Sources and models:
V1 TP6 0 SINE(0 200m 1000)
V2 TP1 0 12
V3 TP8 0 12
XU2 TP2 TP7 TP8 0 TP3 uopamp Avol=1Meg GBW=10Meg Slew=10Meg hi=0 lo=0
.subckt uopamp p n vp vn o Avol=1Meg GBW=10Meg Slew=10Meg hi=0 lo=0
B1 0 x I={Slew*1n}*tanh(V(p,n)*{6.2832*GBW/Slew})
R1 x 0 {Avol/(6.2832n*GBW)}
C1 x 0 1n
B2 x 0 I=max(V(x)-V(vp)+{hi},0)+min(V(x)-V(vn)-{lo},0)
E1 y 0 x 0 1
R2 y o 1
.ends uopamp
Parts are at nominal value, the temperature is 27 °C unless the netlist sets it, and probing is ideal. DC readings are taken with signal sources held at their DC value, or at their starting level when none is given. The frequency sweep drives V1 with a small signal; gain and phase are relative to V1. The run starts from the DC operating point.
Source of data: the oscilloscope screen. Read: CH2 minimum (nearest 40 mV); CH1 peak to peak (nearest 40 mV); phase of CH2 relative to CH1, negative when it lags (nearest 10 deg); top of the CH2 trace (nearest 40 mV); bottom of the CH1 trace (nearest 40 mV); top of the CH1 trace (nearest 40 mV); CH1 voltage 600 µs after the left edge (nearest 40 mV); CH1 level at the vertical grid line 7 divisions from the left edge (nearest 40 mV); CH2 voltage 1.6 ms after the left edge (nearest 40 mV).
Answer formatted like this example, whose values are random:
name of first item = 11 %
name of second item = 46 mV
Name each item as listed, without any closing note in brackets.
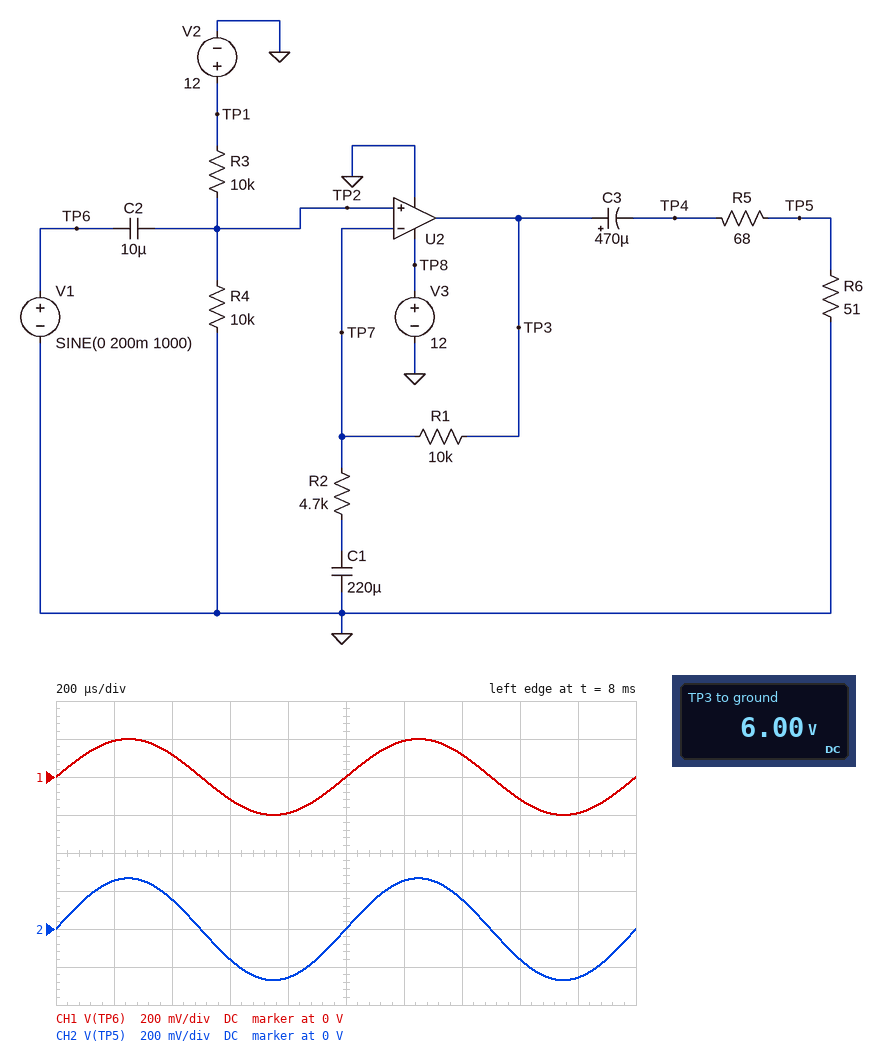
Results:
CH2 minimum = -280 mV
CH1 peak to peak = 400 mV
phase of CH2 relative to CH1, negative when it lags = 0 deg
top of the CH2 trace = 280 mV
bottom of the CH1 trace = -200 mV
top of the CH1 trace = 200 mV
CH1 voltage 600 µs after the left edge = -120 mV
CH1 level at the vertical grid line 7 divisions from the left edge = 120 mV
CH2 voltage 1.6 ms after the left edge = -160 mV
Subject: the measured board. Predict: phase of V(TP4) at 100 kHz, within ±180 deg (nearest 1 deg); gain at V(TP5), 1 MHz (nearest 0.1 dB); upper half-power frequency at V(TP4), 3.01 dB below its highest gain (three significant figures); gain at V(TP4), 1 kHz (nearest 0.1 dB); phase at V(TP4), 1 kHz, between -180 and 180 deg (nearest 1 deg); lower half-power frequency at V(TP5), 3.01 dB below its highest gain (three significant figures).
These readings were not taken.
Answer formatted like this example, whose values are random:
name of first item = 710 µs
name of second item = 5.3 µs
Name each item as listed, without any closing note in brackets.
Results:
phase of V(TP4) at 100 kHz, within ±180 deg = -2 deg
gain at V(TP5), 1 MHz = 2.1 dB
upper half-power frequency at V(TP4), 3.01 dB below its highest gain = 3.17 MHz
gain at V(TP4), 1 kHz = 9.9 dB
phase at V(TP4), 1 kHz, between -180 and 180 deg = 0 deg
lower half-power frequency at V(TP5), 3.01 dB below its highest gain = 4.69 Hz
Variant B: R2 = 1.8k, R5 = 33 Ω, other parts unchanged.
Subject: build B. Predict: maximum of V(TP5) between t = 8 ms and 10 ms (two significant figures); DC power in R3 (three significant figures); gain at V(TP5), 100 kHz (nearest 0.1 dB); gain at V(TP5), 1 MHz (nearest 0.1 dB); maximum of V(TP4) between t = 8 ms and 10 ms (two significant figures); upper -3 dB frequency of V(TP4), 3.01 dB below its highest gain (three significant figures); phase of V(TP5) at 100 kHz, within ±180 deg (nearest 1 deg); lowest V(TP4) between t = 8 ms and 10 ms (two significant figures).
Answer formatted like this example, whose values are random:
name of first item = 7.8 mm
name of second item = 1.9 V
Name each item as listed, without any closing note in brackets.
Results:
maximum of V(TP5) between t = 8 ms and 10 ms = 790 mV
DC power in R3 = 3.60 mW
gain at V(TP5), 100 kHz = 12.0 dB
gain at V(TP5), 1 MHz = 10.4 dB
maximum of V(TP4) between t = 8 ms and 10 ms = 1.3 V
upper -3 dB frequency of V(TP4), 3.01 dB below its highest gain = 1.51 MHz
phase of V(TP5) at 100 kHz, within ±180 deg = -4 deg
lowest V(TP4) between t = 8 ms and 10 ms = -1.3 V
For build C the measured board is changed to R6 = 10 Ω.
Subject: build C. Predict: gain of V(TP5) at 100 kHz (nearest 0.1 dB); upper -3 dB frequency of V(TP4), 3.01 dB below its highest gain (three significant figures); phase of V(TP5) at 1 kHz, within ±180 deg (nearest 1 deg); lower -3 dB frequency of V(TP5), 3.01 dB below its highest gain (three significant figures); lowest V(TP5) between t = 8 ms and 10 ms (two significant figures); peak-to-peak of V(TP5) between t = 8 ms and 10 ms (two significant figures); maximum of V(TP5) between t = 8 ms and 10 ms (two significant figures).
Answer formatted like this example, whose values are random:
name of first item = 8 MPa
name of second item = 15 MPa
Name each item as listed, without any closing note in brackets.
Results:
gain of V(TP5) at 100 kHz = -7.9 dB
upper -3 dB frequency of V(TP4), 3.01 dB below its highest gain = 3.16 MHz
phase of V(TP5) at 1 kHz, within ±180 deg = 0 deg
lower -3 dB frequency of V(TP5), 3.01 dB below its highest gain = 5.88 Hz
lowest V(TP5) between t = 8 ms and 10 ms = -81 mV
peak-to-peak of V(TP5) between t = 8 ms and 10 ms = 160 mV
maximum of V(TP5) between t = 8 ms and 10 ms = 80 mV
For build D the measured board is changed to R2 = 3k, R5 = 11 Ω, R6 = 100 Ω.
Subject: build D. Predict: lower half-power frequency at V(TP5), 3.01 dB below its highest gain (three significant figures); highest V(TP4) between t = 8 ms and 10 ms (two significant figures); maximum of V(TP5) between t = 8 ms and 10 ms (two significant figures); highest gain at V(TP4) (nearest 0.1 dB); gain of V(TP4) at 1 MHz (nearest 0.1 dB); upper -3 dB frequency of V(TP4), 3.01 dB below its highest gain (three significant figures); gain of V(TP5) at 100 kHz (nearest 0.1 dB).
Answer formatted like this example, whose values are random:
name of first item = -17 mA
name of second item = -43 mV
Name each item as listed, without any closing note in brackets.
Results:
lower half-power frequency at V(TP5), 3.01 dB below its highest gain = 4.85 Hz
highest V(TP4) between t = 8 ms and 10 ms = 860 mV
maximum of V(TP5) between t = 8 ms and 10 ms = 780 mV
highest gain at V(TP4) = 12.7 dB
gain of V(TP4) at 1 MHz = 12.0 dB
upper -3 dB frequency of V(TP4), 3.01 dB below its highest gain = 2.29 MHz
gain of V(TP5) at 100 kHz = 11.8 dB
